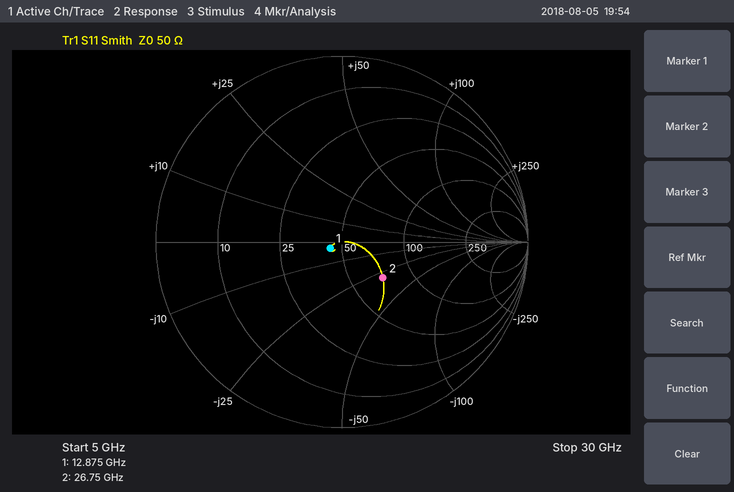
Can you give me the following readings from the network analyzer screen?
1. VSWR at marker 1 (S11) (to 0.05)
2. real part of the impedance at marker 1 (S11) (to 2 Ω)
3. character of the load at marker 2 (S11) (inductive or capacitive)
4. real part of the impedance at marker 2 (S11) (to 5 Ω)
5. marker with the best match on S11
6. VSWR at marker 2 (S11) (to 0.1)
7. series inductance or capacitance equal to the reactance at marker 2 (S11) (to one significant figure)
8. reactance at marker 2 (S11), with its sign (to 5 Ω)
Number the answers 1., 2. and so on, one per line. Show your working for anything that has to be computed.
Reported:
1. 1.15
2. 44 Ω
3. capacitive
4. 70 Ω
5. marker 1
6. 1.8
7. C = 1/(2π × 26.75 GHz × 30 Ω) ≈ 198 fF, so 200 fF to one significant figure
8. -30 Ω
